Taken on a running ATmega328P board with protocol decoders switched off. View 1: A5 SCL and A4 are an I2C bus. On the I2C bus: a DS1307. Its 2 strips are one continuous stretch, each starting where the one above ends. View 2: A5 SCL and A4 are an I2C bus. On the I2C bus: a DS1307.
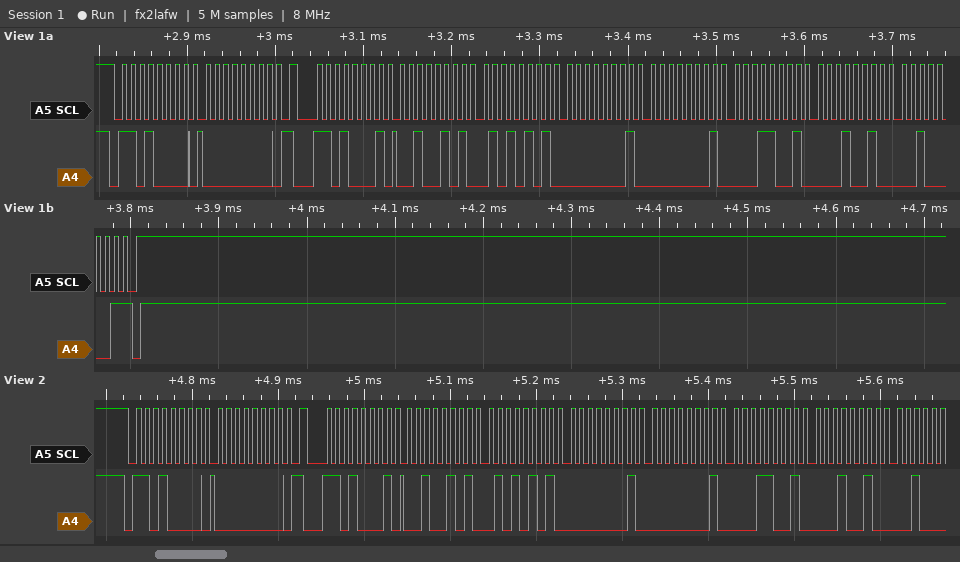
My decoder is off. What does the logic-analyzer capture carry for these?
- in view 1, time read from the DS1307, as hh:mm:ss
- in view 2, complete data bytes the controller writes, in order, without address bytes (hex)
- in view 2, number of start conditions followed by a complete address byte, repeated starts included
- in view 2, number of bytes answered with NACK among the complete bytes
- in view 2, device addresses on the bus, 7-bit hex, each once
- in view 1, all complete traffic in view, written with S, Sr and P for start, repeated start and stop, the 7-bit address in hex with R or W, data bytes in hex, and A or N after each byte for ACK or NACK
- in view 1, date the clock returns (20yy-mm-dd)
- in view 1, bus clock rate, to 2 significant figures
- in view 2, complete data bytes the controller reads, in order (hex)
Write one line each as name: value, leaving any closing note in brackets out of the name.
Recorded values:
in view 1, time read from the DS1307, as hh:mm:ss: 01:55:25
in view 2, complete data bytes the controller writes, in order, without address bytes: 00
in view 2, number of start conditions followed by a complete address byte, repeated starts included: 2
in view 2, number of bytes answered with NACK among the complete bytes: 0
in view 2, device addresses on the bus, 7-bit hex, each once: 0x68
in view 1, all complete traffic in view, written with S, Sr and P for start, repeated start and stop, the 7-bit address in hex with R or W, data bytes in hex, and A or N after each byte for ACK or NACK: S 68W A 00 A Sr 68R A 25 A 55 A 01 A 01 A 19 A 12 A 21 N P
in view 1, date the clock returns: 2021-12-19
in view 1, bus clock rate, to 2 significant figures: 100 kHz
in view 2, complete data bytes the controller reads, in order: 25 55 01 01 19 12
